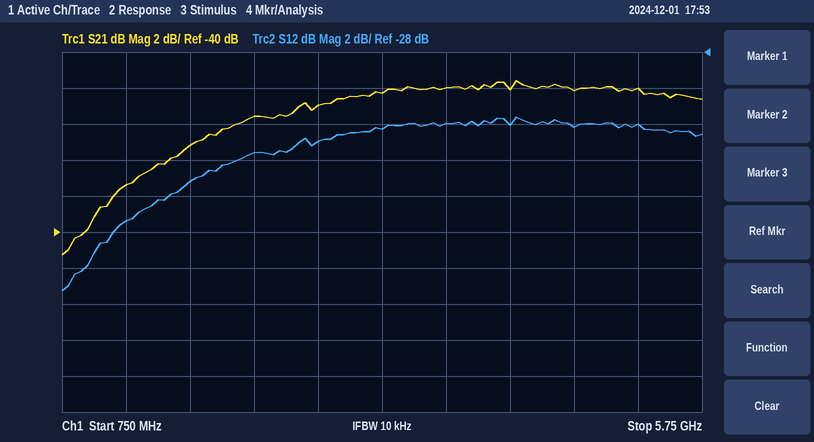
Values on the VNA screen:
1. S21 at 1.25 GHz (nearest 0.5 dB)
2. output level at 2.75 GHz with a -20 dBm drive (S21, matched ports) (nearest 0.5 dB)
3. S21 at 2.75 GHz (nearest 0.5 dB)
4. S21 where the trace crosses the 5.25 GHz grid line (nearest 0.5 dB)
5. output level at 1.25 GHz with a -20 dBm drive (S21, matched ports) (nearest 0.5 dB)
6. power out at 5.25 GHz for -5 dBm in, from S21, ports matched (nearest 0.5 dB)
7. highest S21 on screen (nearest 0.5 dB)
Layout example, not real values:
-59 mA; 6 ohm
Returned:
-37.5 dB; -53.0 dBm; -33.0 dB; -32.0 dB; -57.5 dBm; -37.0 dBm; -31.5 dB
